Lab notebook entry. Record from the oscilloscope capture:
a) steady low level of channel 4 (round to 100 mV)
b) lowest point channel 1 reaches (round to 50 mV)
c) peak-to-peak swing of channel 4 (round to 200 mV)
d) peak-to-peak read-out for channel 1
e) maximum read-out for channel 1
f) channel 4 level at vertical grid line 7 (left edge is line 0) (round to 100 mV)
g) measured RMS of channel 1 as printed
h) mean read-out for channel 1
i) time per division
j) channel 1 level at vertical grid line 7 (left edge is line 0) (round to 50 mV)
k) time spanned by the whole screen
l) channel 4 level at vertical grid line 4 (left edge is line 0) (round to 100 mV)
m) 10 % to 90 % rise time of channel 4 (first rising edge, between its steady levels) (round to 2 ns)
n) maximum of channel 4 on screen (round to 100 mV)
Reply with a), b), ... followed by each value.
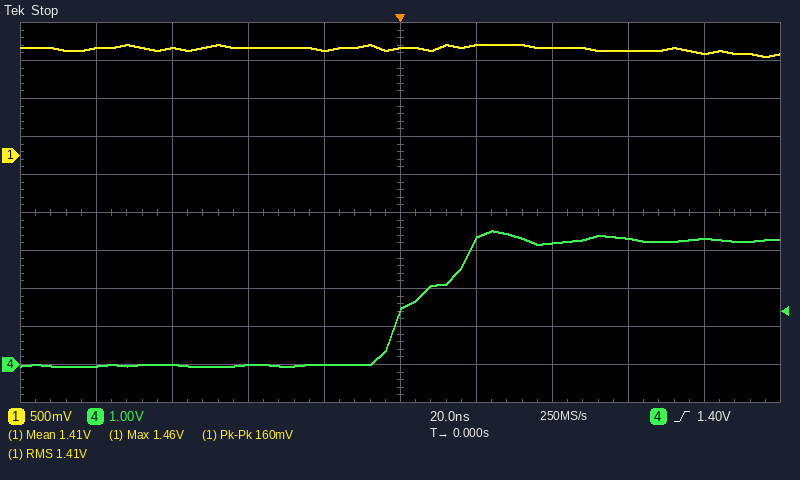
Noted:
a) 0.0 V
b) 1.30 V
c) 3.6 V
d) 160 mV
e) 1.46 V
f) 3.2 V
g) 1.41 V
h) 1.41 V
i) 20 ns
j) 1.40 V
k) 200 ns
l) 0.0 V
m) 22 ns
n) 3.5 V
